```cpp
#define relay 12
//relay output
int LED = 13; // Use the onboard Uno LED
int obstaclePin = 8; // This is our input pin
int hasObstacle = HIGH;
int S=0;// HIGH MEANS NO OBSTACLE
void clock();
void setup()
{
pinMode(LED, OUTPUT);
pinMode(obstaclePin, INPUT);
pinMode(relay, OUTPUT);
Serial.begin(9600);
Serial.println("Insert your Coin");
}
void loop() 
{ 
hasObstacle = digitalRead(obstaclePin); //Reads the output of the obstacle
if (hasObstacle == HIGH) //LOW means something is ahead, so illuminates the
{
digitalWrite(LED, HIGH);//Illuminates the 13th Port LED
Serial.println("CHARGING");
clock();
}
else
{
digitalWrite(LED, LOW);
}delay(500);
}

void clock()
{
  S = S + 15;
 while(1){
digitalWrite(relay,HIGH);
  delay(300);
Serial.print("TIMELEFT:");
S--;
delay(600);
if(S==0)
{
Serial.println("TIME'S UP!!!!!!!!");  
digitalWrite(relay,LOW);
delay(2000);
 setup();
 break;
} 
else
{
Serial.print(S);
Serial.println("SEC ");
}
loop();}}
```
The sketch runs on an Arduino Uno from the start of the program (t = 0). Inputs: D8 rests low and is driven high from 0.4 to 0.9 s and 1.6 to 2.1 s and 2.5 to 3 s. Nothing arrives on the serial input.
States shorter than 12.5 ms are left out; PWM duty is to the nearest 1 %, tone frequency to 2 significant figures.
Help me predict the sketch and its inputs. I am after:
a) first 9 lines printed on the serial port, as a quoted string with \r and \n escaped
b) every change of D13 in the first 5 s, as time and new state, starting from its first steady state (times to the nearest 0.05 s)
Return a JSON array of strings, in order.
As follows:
["\"Insert your Coin\\r\\nCHARGING\\r\\nTIMELEFT:14SEC \\r\\nTIMELEFT:13SEC \\r\\nCHARGING\\r\\nTIMELEFT:27SEC \\r\\nTIMELEFT:26SEC \\r\\nTIMELEFT:25SEC \\r\\nTIMELEFT:24SEC \\r\\n\"", "0 s low; 0.5 s high; 1.4 s low; 2.8 s high; 3.7 s low"]
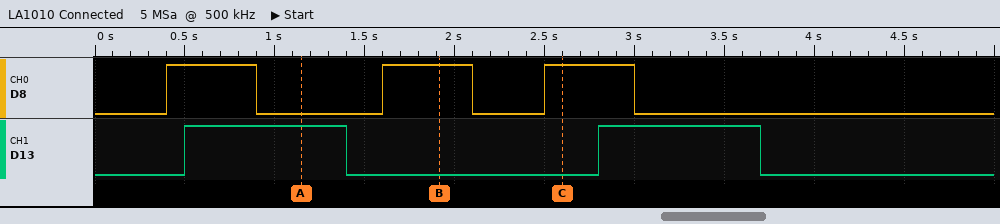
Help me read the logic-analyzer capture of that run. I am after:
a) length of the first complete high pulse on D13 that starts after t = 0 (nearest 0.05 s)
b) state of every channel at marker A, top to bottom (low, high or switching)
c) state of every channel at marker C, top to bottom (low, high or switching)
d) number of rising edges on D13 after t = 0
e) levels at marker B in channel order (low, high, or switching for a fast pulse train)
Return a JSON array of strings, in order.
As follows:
["0.90 s", "D8 low, D13 high", "D8 high, D13 low", "2", "D8 high, D13 low"]
